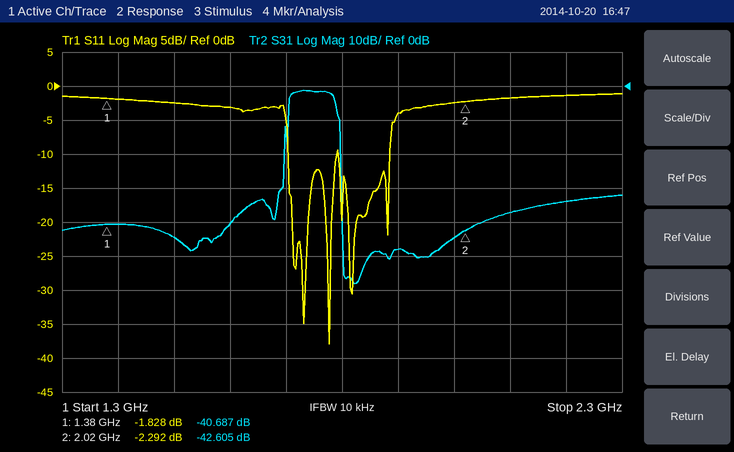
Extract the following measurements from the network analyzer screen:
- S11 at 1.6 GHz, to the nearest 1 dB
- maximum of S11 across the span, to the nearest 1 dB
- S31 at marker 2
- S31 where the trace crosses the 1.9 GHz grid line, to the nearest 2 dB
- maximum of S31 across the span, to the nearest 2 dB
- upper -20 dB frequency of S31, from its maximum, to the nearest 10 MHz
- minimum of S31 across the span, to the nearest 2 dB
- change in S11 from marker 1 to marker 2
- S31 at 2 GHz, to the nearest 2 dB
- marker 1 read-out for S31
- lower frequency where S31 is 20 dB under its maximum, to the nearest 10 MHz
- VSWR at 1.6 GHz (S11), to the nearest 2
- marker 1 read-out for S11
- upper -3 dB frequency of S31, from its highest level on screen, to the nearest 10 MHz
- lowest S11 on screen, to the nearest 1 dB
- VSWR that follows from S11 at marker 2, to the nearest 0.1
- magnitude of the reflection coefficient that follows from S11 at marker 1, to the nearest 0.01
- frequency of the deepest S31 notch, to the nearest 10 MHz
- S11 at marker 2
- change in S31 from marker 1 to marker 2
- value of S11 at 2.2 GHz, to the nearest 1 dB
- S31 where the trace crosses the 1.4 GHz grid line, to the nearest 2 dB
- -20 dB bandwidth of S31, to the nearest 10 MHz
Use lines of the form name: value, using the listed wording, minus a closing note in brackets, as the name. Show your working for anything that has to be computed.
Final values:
S11 at 1.6 GHz, to the nearest 1 dB: -3 dB
maximum of S11 across the span, to the nearest 1 dB: -1 dB
S31 at marker 2: -42.605 dB
S31 where the trace crosses the 1.9 GHz grid line, to the nearest 2 dB: -48 dB
maximum of S31 across the span, to the nearest 2 dB: -2 dB
upper -20 dB frequency of S31, from its maximum, to the nearest 10 MHz: 1.80 GHz
minimum of S31 across the span, to the nearest 2 dB: -58 dB
change in S11 from marker 1 to marker 2: -2.292 − (-1.828) = -0.464 dB
S31 at 2 GHz, to the nearest 2 dB: -44 dB
marker 1 read-out for S31: -40.687 dB
lower frequency where S31 is 20 dB under its maximum, to the nearest 10 MHz: 1.70 GHz
VSWR at 1.6 GHz (S11), to the nearest 2: |Γ| = 10^(-3/20) = 0.7079; VSWR = (1 + 0.7079)/(1 − 0.7079) ≈ 6
marker 1 read-out for S11: -1.828 dB
upper -3 dB frequency of S31, from its highest level on screen, to the nearest 10 MHz: 1.79 GHz
lowest S11 on screen, to the nearest 1 dB: -38 dB
VSWR that follows from S11 at marker 2, to the nearest 0.1: (1 + 0.7681)/(1 − 0.7681) ≈ 7.6
magnitude of the reflection coefficient that follows from S11 at marker 1, to the nearest 0.01: 10^(-1.828/20) ≈ 0.81
frequency of the deepest S31 notch, to the nearest 10 MHz: 1.82 GHz
S11 at marker 2: -2.292 dB
change in S31 from marker 1 to marker 2: -42.605 − (-40.687) = -1.918 dB
value of S11 at 2.2 GHz, to the nearest 1 dB: -1 dB
S31 where the trace crosses the 1.4 GHz grid line, to the nearest 2 dB: -40 dB
-20 dB bandwidth of S31, to the nearest 10 MHz: 1.80 GHz − 1.70 GHz = 100 MHz
